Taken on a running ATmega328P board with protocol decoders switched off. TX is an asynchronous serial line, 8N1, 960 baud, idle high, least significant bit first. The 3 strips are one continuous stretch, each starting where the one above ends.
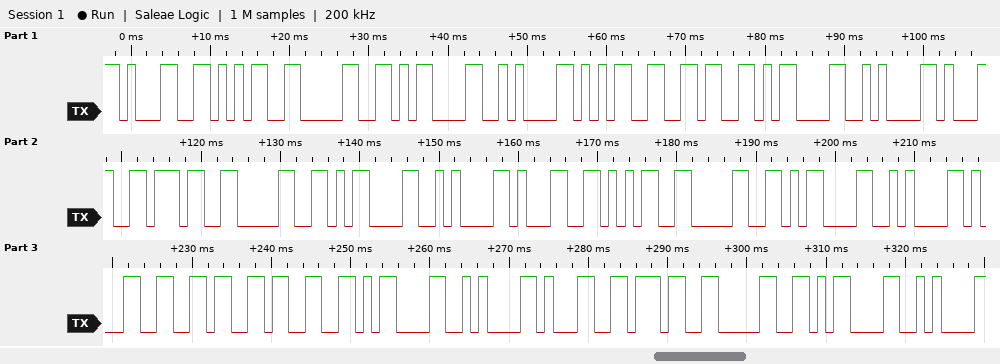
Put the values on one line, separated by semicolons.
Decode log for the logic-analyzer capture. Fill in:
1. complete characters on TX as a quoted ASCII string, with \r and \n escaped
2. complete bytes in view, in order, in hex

"150\r\n56\r\n170\r\n150\r\n163\r\n170\r\n"; 31 35 30 0D 0A 35 36 0D 0A 31 37 30 0D 0A 31 35 30 0D 0A 31 36 33 0D 0A 31 37 30 0D 0A
